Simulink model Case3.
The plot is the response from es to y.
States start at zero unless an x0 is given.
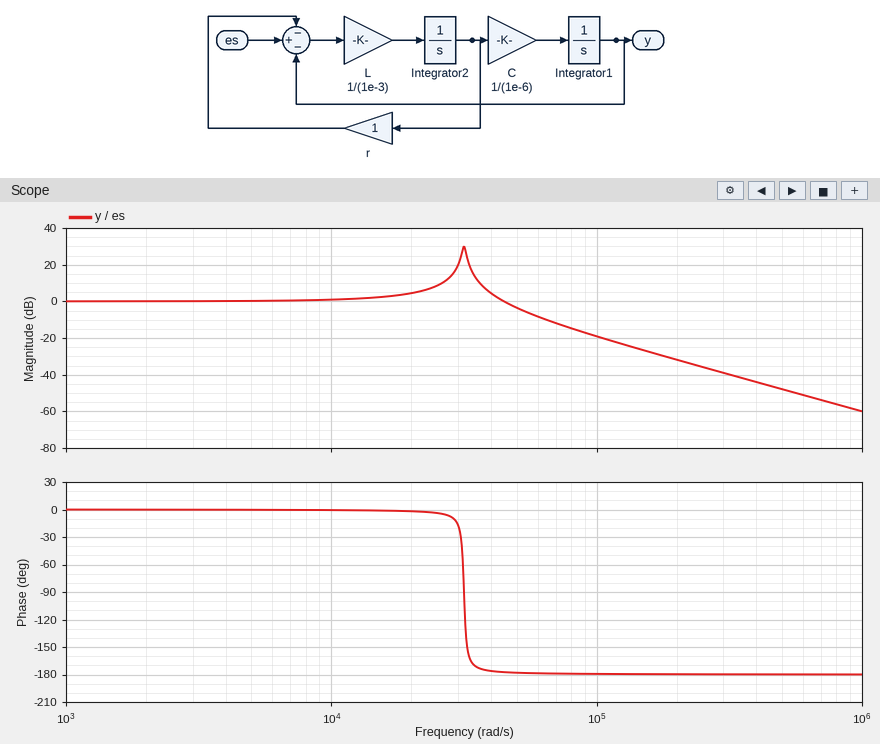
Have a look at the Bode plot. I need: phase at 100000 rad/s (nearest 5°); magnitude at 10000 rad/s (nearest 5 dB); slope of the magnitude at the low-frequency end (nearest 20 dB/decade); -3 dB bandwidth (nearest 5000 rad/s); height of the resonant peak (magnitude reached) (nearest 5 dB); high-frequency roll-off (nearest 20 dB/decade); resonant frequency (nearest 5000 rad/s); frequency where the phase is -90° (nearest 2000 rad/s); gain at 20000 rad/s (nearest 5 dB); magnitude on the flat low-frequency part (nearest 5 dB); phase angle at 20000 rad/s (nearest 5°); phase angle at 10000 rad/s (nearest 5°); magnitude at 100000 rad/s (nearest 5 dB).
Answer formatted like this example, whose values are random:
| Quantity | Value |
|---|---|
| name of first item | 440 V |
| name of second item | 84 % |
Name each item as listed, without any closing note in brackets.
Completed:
| Quantity | Value |
|---|---|
| phase at 100000 rad/s | -180° |
| magnitude at 10000 rad/s | 0 dB |
| slope of the magnitude at the low-frequency end | 0 dB/decade |
| -3 dB bandwidth | 50000 rad/s |
| height of the resonant peak (magnitude reached) | 30 dB |
| high-frequency roll-off | -40 dB/decade |
| resonant frequency | 30000 rad/s |
| frequency where the phase is -90° | 32000 rad/s |
| gain at 20000 rad/s | 5 dB |
| magnitude on the flat low-frequency part | 0 dB |
| phase angle at 20000 rad/s | 0° |
| phase angle at 10000 rad/s | 0° |
| magnitude at 100000 rad/s | -20 dB |
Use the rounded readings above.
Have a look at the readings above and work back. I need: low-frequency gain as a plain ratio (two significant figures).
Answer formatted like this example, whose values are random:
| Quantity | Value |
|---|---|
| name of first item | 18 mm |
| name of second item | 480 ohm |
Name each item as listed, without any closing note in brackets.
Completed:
| Quantity | Value |
|---|---|
| low-frequency gain as a plain ratio | 1.0 |
